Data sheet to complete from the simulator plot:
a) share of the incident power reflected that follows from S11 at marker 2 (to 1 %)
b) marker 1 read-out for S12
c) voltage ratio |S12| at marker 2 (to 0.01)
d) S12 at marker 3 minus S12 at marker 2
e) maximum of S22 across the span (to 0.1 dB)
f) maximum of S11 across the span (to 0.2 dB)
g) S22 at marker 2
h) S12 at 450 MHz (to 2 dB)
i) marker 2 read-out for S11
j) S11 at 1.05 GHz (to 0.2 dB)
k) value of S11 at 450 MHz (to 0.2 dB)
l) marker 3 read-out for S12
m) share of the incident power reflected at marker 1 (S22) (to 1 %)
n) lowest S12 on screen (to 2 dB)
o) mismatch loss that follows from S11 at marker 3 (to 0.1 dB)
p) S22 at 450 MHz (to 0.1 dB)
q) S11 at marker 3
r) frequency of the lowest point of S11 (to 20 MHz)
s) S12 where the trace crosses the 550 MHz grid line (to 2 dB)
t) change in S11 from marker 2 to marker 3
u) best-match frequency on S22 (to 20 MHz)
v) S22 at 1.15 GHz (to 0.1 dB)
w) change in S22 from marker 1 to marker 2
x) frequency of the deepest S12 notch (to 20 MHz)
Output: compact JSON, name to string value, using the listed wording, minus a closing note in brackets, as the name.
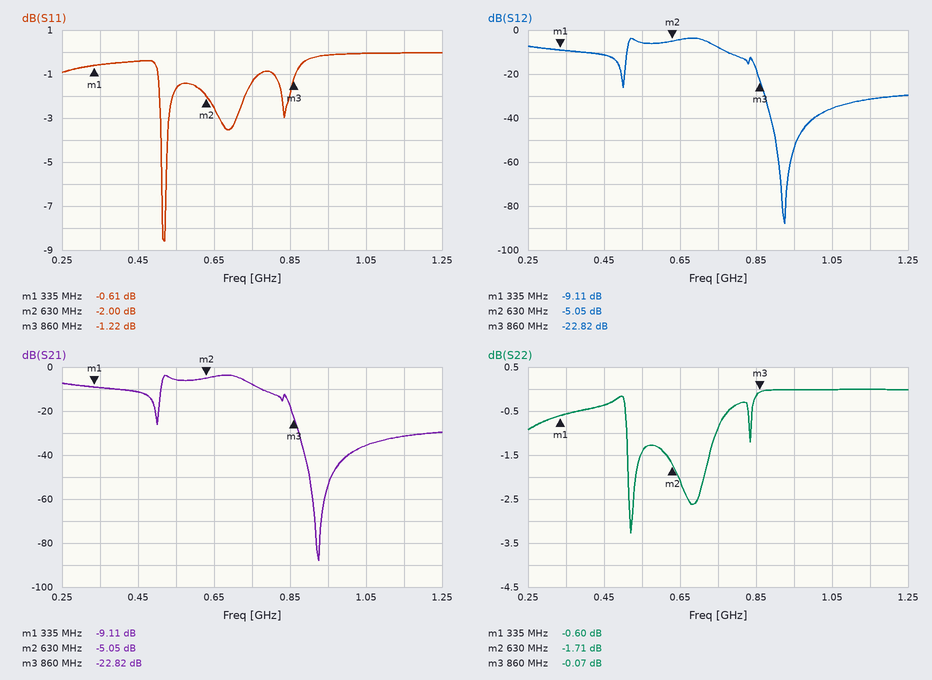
{"share of the incident power reflected that follows from S11 at marker 2": "63 %", "marker 1 read-out for S12": "-9.11 dB", "voltage ratio |S12| at marker 2": "0.56", "S12 at marker 3 minus S12 at marker 2": "-17.77 dB", "maximum of S22 across the span": "0.0 dB", "maximum of S11 across the span": "0.0 dB", "S22 at marker 2": "-1.71 dB", "S12 at 450 MHz": "-12 dB", "marker 2 read-out for S11": "-2.00 dB", "S11 at 1.05 GHz": "0.0 dB", "value of S11 at 450 MHz": "-0.4 dB", "marker 3 read-out for S12": "-22.82 dB", "share of the incident power reflected at marker 1 (S22)": "87 %", "lowest S12 on screen": "-88 dB", "mismatch loss that follows from S11 at marker 3": "6.1 dB", "S22 at 450 MHz": "-0.4 dB", "S11 at marker 3": "-1.22 dB", "frequency of the lowest point of S11": "520 MHz", "S12 where the trace crosses the 550 MHz grid line": "-6 dB", "change in S11 from marker 2 to marker 3": "0.78 dB", "best-match frequency on S22": "520 MHz", "S22 at 1.15 GHz": "0.0 dB", "change in S22 from marker 1 to marker 2": "-1.11 dB", "frequency of the deepest S12 notch": "920 MHz"}
